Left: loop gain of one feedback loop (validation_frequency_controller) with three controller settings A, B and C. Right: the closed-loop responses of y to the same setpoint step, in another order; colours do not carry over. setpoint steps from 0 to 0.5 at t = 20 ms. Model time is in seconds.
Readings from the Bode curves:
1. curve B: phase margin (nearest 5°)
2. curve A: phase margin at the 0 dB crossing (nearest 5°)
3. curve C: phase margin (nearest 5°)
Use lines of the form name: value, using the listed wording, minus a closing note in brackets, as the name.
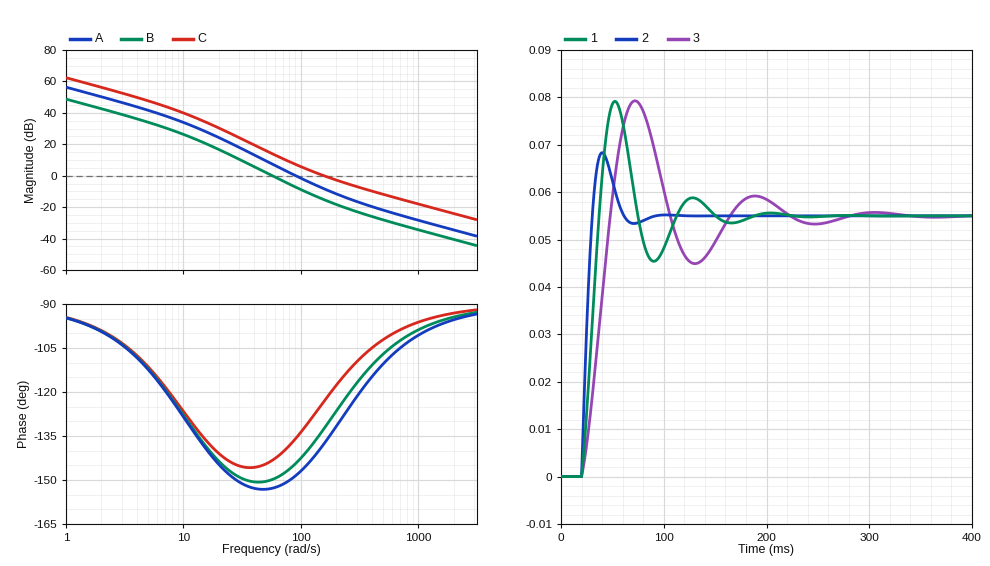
curve B: phase margin: 30°
curve A: phase margin at the 0 dB crossing: 30°
curve C: phase margin: 55°
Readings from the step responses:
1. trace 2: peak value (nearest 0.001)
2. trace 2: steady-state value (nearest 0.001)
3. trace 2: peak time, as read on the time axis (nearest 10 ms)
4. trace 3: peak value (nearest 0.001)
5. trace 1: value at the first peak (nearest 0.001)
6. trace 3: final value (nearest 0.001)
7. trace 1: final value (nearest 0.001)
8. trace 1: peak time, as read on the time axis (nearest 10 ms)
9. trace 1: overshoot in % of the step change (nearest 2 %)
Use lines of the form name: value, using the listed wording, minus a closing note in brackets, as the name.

trace 2: peak value: 0.068
trace 2: steady-state value: 0.055
trace 2: peak time, as read on the time axis: 40 ms
trace 3: peak value: 0.079
trace 1: value at the first peak: 0.079
trace 3: final value: 0.055
trace 1: final value: 0.055
trace 1: peak time, as read on the time axis: 50 ms
trace 1: overshoot in % of the step change: 44 %
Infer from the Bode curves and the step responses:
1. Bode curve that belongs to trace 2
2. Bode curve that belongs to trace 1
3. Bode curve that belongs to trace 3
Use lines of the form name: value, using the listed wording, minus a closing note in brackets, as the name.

Bode curve that belongs to trace 2: C
Bode curve that belongs to trace 1: A
Bode curve that belongs to trace 3: B
